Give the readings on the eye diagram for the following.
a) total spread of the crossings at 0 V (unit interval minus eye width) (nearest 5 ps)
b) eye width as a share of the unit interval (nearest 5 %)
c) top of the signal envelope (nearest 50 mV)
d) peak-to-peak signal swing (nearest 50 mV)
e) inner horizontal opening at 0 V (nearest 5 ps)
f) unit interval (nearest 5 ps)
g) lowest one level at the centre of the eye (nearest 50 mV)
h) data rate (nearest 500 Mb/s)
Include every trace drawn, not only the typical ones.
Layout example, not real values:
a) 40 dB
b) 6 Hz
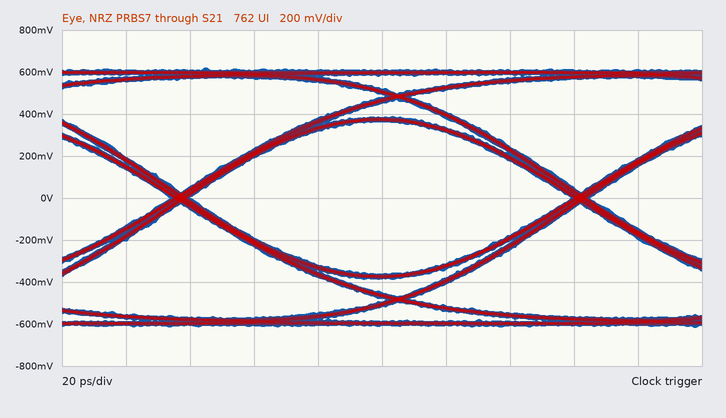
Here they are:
a) 5 ps
b) 95 %
c) 600 mV
d) 1.25 V
e) 120 ps
f) 125 ps
g) 350 mV
h) 8.0 Gb/s
